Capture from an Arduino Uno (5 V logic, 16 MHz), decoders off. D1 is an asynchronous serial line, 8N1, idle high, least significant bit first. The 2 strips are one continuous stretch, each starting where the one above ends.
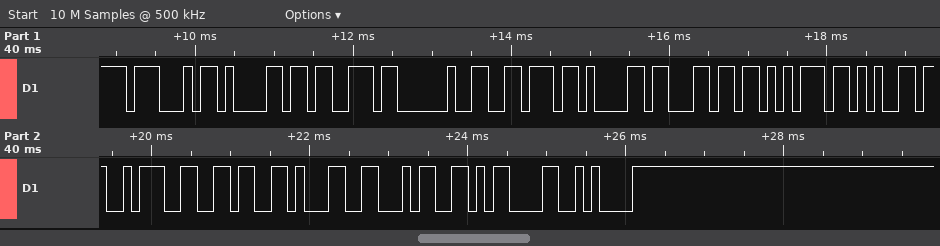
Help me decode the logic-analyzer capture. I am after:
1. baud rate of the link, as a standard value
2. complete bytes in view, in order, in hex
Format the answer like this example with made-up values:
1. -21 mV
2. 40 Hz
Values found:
1. 9600 baud
2. 47 61 73 20 76 61 6C 75 65 3A 36 31 34 0D 0A
